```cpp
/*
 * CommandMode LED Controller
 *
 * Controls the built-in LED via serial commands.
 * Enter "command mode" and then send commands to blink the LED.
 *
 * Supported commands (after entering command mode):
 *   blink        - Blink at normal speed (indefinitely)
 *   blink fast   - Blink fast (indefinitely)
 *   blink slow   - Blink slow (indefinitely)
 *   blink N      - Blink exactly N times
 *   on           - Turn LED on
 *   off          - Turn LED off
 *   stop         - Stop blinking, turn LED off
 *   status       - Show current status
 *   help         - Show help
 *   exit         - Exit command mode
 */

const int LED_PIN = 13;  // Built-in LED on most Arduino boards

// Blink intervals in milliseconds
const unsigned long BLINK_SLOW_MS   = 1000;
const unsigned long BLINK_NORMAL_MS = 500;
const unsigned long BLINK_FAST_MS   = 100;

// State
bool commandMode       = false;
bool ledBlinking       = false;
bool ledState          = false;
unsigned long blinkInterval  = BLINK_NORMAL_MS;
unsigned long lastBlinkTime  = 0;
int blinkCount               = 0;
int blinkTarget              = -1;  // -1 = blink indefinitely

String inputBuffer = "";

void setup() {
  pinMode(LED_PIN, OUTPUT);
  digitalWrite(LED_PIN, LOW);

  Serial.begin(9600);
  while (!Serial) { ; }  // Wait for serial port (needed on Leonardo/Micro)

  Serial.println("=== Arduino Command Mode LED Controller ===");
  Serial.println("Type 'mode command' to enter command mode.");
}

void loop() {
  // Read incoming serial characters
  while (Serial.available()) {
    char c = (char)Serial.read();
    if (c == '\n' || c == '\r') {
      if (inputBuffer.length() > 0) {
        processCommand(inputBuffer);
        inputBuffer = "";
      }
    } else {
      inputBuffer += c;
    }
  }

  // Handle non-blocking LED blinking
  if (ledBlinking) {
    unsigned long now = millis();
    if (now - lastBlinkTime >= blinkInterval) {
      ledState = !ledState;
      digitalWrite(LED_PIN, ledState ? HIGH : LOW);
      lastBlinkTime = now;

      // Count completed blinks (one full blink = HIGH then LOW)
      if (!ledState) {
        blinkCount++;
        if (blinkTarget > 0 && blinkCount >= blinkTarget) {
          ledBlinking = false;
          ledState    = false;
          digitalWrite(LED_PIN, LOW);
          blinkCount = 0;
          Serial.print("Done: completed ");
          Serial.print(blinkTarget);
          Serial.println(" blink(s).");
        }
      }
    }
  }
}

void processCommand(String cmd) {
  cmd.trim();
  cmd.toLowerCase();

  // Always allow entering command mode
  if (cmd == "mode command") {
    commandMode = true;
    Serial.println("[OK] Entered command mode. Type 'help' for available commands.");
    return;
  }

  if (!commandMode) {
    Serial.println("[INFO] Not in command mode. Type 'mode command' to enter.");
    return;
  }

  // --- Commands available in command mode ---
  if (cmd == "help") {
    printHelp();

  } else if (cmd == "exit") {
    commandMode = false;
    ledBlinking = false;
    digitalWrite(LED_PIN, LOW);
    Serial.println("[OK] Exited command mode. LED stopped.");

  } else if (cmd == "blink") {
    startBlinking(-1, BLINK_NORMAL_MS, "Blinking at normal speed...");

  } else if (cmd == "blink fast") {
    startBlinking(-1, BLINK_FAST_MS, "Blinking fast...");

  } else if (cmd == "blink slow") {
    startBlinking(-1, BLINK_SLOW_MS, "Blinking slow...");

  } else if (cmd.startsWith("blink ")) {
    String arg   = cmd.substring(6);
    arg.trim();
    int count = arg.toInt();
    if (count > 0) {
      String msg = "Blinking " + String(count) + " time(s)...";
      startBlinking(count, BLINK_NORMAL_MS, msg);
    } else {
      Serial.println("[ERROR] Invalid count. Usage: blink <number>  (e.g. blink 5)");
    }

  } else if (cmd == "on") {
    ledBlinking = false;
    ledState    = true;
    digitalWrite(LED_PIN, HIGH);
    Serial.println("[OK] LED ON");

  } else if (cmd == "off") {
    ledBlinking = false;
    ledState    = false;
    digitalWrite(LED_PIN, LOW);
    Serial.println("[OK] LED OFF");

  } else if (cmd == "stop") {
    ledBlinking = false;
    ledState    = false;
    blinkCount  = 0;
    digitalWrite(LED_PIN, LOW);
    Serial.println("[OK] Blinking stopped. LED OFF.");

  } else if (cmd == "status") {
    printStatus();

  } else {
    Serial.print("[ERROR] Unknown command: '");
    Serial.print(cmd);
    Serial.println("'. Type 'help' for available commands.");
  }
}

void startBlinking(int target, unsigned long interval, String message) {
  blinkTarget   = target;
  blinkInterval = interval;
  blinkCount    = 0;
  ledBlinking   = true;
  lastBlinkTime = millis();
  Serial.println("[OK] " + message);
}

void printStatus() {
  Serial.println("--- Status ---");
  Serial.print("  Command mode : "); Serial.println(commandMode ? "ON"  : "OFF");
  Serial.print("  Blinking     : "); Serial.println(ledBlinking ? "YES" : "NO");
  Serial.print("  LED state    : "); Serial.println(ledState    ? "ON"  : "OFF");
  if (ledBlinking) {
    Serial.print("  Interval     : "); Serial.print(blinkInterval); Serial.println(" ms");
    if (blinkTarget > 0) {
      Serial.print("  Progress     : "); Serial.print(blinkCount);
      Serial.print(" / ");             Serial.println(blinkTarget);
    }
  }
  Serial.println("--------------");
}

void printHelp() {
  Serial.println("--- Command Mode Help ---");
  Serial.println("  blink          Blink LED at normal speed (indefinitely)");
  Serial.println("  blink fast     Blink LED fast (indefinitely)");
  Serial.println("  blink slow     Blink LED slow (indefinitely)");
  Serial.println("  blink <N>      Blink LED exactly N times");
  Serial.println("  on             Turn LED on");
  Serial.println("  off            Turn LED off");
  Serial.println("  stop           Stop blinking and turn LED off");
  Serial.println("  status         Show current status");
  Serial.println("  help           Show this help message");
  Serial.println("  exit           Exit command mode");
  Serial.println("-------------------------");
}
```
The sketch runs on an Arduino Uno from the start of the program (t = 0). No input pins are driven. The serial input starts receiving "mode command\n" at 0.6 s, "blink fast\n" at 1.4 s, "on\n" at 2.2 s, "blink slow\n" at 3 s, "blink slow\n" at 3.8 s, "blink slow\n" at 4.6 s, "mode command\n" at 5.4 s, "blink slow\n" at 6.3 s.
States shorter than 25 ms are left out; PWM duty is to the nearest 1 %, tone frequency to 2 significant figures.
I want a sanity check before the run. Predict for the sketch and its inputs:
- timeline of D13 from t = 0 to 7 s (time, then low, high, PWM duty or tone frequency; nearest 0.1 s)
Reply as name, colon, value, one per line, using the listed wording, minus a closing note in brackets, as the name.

timeline of D13 from t = 0 to 7 s: 0 s low; 1.5 s high; 1.6 s low; 1.7 s high; 1.8 s low; 1.9 s high; 2 s low; 2.1 s high; 5.6 s low
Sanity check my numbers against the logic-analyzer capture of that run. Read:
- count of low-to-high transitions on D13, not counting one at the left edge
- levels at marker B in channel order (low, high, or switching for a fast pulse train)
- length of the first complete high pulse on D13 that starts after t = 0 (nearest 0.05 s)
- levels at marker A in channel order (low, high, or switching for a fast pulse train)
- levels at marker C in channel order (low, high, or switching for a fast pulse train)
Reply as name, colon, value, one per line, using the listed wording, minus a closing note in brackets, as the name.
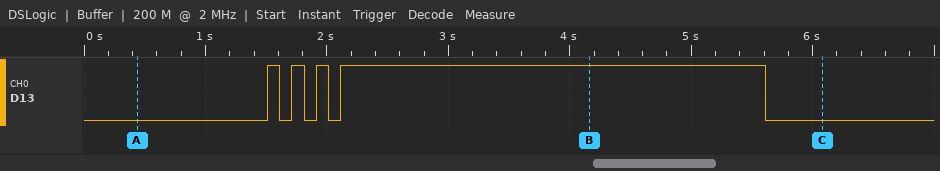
count of low-to-high transitions on D13, not counting one at the left edge: 4
levels at marker B in channel order: D13 high
length of the first complete high pulse on D13 that starts after t = 0: 0.10 s
levels at marker A in channel order: D13 low
levels at marker C in channel order: D13 low
